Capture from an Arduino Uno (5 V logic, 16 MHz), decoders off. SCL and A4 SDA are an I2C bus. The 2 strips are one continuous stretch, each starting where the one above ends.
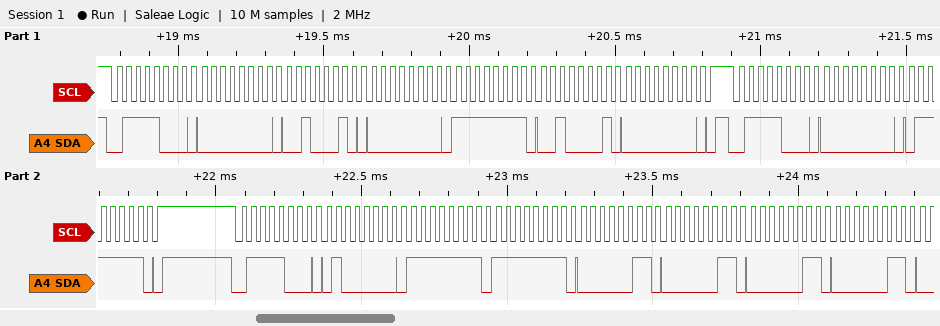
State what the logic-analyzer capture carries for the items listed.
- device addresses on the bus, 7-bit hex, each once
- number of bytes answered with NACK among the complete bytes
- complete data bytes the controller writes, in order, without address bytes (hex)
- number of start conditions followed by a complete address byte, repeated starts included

0x3C
0
00 22 00 FF 21 00 00 7F 40 FF FF 03 03 03 03
3
